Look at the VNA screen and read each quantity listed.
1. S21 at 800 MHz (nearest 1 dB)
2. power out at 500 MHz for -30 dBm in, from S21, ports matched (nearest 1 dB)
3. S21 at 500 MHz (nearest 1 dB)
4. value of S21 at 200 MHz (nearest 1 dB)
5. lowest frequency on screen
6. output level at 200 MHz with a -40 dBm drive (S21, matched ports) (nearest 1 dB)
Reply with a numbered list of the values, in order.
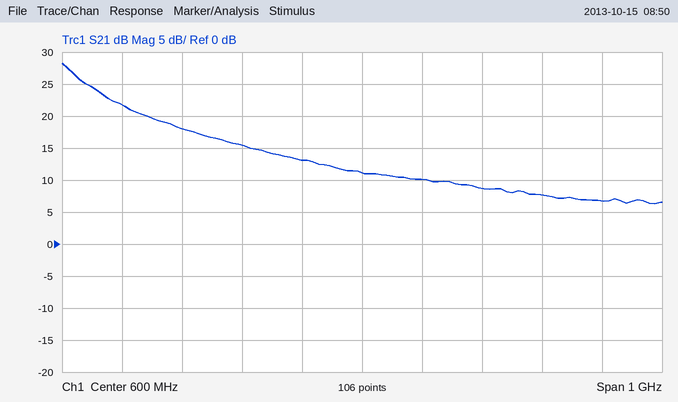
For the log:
1. 9 dB
2. -17 dBm
3. 13 dB
4. 22 dB
5. 100 MHz
6. -18 dBm
